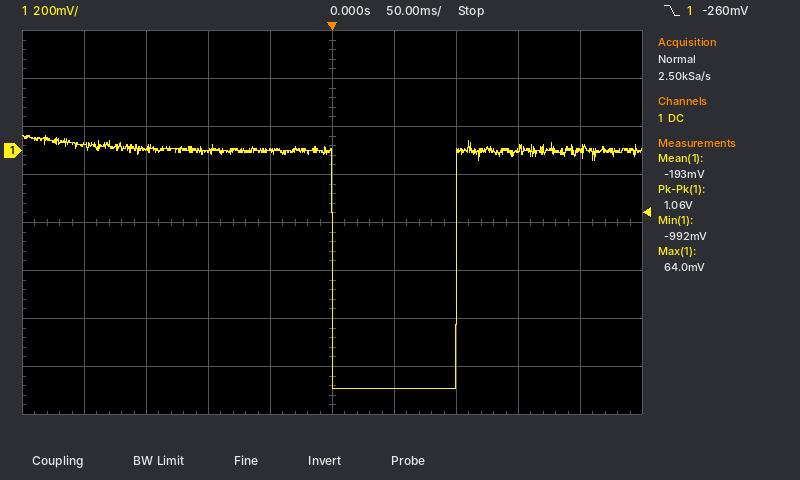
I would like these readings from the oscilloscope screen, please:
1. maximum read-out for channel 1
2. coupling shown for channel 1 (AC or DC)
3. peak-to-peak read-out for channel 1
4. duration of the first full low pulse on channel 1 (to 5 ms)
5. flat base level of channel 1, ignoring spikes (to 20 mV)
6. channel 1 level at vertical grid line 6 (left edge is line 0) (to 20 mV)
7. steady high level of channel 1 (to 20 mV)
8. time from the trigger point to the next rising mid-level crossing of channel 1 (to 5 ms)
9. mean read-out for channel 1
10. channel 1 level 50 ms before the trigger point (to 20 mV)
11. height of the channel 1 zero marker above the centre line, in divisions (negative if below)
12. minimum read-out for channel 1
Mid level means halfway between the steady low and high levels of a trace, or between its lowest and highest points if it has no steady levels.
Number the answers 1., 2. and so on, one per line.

1. 64.0 mV
2. DC
3. 1.06 V
4. 100 ms
5. -1.00 V
6. -1.00 V
7. 0 mV
8. 100 ms
9. -193 mV
10. 0 mV
11. +1.5 div
12. -992 mV
